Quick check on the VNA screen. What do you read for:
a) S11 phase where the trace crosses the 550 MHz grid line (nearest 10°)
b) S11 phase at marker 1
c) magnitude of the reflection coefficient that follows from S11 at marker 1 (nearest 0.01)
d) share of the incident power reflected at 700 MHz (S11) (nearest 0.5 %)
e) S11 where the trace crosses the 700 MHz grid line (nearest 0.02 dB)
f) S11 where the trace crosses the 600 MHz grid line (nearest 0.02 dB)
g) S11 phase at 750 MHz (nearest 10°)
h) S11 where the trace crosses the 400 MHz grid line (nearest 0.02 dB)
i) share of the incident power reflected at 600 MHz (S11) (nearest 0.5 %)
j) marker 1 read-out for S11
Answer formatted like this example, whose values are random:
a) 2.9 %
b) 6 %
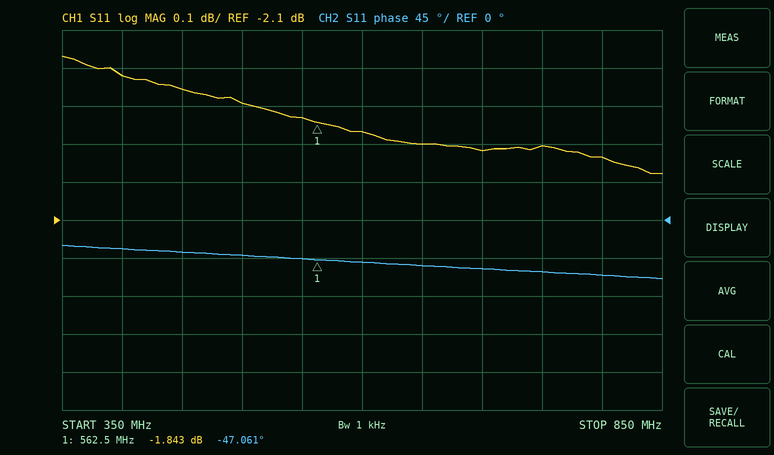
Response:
a) -50°
b) -47.061°
c) 0.81
d) 64.5 %
e) -1.92 dB
f) -1.86 dB
g) -60°
h) -1.72 dB
i) 65.0 %
j) -1.843 dB
